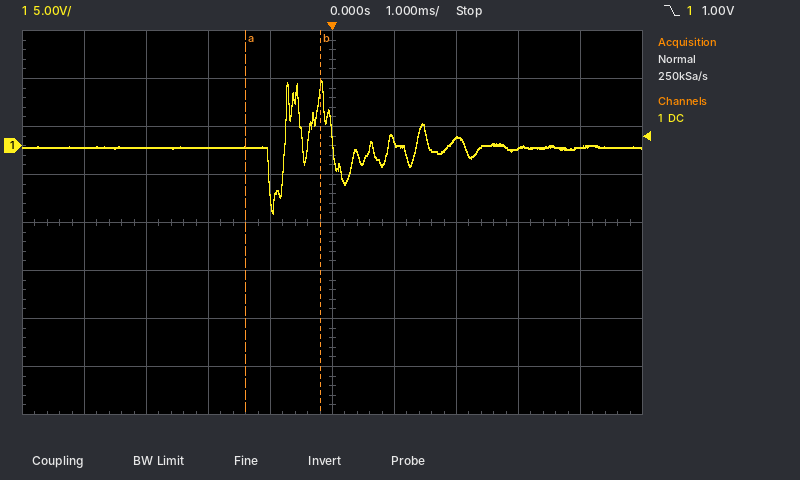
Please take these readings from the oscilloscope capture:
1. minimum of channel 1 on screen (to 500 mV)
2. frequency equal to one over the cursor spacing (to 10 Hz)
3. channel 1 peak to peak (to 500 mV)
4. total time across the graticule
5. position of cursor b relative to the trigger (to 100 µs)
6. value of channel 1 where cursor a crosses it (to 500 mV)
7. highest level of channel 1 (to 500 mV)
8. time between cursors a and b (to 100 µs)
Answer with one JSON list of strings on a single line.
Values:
["-7.0 V", "830 Hz", "14.0 V", "10 ms", "-200 µs", "0.0 V", "7.0 V", "1.2 ms"]
